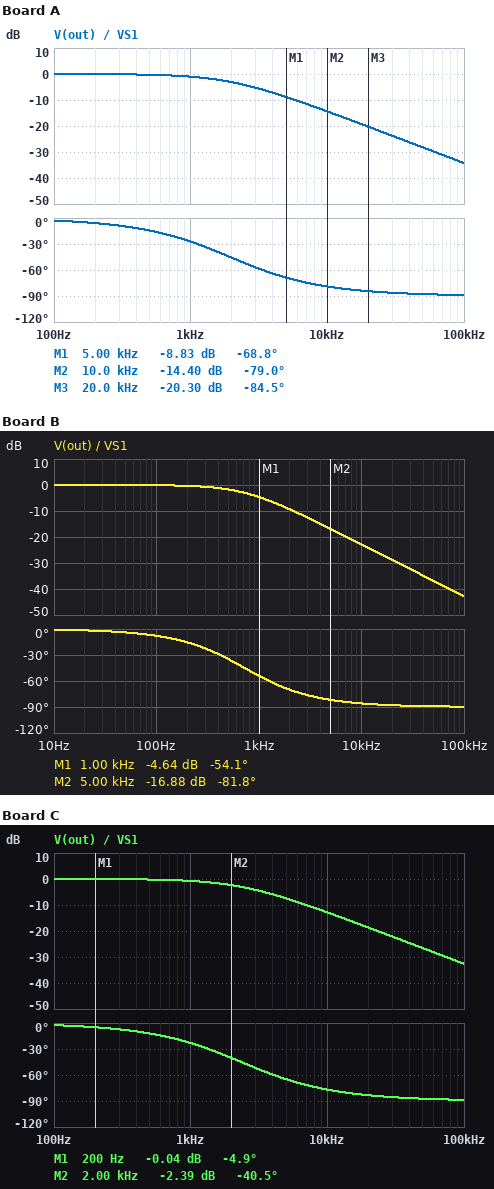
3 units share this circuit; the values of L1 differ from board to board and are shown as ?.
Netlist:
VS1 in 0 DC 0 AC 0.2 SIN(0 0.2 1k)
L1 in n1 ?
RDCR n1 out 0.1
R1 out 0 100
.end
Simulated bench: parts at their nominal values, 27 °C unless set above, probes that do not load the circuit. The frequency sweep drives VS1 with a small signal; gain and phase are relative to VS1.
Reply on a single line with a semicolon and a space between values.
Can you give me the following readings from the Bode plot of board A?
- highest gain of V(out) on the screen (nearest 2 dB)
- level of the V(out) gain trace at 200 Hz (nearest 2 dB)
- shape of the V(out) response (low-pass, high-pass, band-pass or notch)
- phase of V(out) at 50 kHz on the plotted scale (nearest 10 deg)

0 dB; 0 dB; low-pass; -90 deg
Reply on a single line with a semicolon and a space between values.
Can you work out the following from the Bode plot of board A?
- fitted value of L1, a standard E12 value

8.2 mH
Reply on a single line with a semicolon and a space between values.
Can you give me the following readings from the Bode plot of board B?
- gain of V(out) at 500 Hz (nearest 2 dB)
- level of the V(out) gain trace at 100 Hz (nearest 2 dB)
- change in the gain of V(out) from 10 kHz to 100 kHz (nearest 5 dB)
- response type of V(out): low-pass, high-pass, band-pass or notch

-2 dB; 0 dB; -20 dB; low-pass
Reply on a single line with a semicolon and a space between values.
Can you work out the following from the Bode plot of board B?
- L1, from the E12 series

22 mH
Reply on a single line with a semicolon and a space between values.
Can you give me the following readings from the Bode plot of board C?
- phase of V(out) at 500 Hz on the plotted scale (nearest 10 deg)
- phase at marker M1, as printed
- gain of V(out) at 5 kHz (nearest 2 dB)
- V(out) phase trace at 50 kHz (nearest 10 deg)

-10 deg; -4.9 deg; -8 dB; -90 deg
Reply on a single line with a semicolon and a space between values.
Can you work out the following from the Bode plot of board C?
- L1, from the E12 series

6.8 mH
